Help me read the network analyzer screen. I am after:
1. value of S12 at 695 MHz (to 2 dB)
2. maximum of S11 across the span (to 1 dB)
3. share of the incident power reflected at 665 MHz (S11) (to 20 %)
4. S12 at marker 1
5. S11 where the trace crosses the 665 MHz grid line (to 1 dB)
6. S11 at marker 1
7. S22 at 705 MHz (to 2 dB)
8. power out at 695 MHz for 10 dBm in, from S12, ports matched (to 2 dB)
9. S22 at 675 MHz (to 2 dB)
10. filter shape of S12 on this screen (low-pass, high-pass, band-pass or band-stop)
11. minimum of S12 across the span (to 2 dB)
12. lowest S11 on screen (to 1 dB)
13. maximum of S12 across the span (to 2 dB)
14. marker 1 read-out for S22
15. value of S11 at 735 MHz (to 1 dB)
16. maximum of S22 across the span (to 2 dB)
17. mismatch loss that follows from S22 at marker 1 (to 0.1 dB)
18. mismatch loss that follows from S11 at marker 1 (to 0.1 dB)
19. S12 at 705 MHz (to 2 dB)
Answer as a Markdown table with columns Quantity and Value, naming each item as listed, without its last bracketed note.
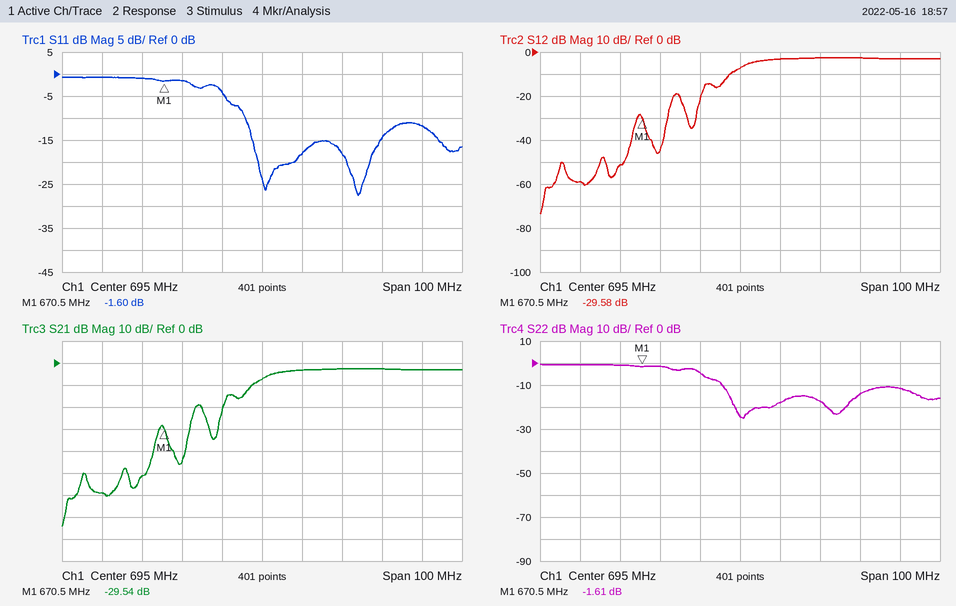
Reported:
| Quantity | Value |
|---|---|
| value of S12 at 695 MHz | -8 dB |
| maximum of S11 across the span | -1 dB |
| share of the incident power reflected at 665 MHz (S11) | 80 % |
| S12 at marker 1 | -29.58 dB |
| S11 where the trace crosses the 665 MHz grid line | -1 dB |
| S11 at marker 1 | -1.60 dB |
| S22 at 705 MHz | -18 dB |
| power out at 695 MHz for 10 dBm in, from S12, ports matched | 2 dBm |
| S22 at 675 MHz | -2 dB |
| filter shape of S12 on this screen | high-pass |
| minimum of S12 across the span | -74 dB |
| lowest S11 on screen | -28 dB |
| maximum of S12 across the span | -2 dB |
| marker 1 read-out for S22 | -1.61 dB |
| value of S11 at 735 MHz | -12 dB |
| maximum of S22 across the span | 0 dB |
| mismatch loss that follows from S22 at marker 1 | 5.1 dB |
| mismatch loss that follows from S11 at marker 1 | 5.1 dB |
| S12 at 705 MHz | -4 dB |
